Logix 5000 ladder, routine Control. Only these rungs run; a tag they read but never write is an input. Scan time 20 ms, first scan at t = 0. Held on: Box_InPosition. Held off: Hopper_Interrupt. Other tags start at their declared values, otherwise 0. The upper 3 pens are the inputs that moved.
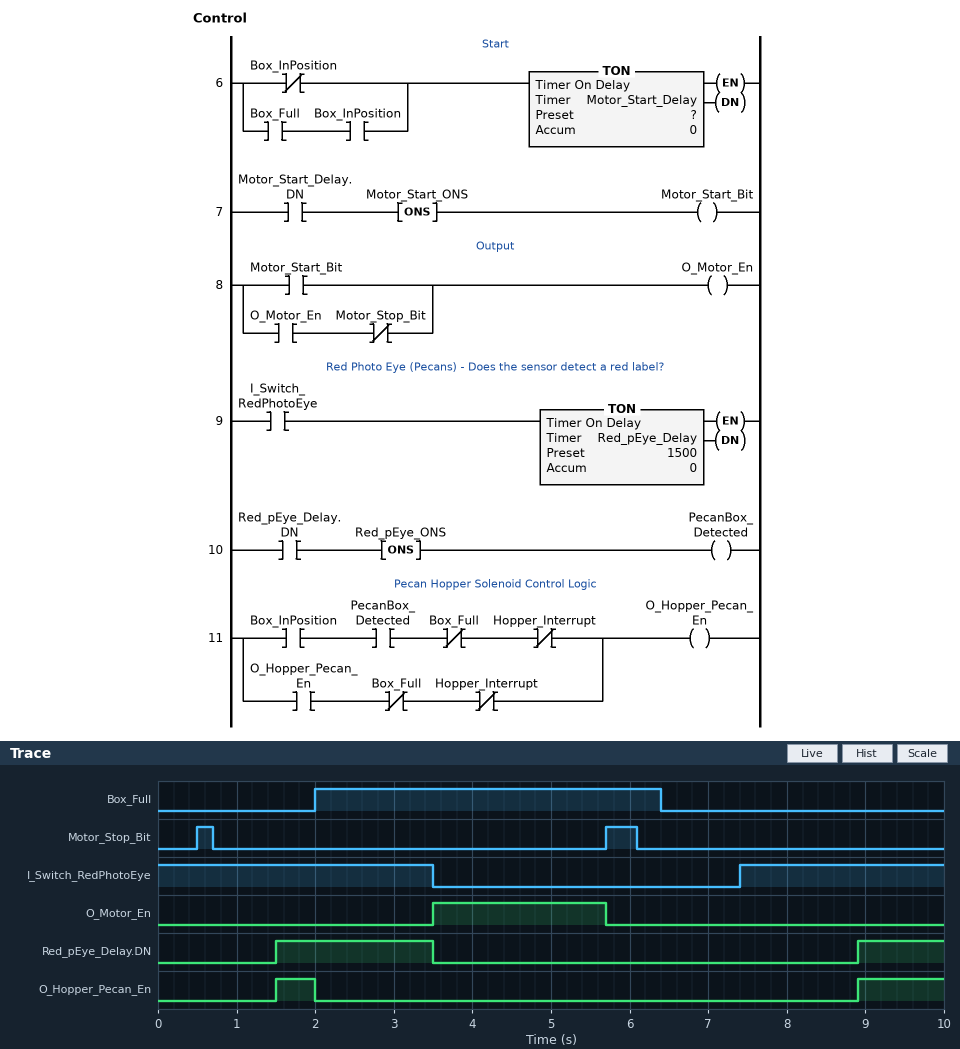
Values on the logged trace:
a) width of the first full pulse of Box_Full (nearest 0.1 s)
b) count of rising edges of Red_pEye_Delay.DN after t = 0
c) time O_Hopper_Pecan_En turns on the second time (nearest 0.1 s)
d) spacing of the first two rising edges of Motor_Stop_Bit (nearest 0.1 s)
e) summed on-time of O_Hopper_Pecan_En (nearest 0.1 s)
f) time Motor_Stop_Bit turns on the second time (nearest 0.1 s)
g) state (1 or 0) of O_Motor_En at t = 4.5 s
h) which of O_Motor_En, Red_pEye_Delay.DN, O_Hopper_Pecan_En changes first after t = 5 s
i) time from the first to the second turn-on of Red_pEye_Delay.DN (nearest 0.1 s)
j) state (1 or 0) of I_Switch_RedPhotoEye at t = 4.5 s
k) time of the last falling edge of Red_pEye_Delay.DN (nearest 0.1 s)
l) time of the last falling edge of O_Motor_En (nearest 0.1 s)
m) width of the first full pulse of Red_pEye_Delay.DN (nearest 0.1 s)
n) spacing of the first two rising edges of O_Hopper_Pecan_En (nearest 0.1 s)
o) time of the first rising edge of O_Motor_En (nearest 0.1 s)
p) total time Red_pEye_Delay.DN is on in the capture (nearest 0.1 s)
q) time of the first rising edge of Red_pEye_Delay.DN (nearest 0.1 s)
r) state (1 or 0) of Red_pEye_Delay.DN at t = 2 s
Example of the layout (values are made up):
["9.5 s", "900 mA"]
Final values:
["4.4 s", "2", "8.9 s", "5.2 s", "1.6 s", "5.7 s", "1", "O_Motor_En", "7.4 s", "0", "3.5 s", "5.7 s", "2.0 s", "7.4 s", "3.5 s", "3.1 s", "1.5 s", "1"]
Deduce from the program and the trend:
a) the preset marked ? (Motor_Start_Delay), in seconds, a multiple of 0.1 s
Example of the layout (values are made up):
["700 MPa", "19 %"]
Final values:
["1.5 s"]
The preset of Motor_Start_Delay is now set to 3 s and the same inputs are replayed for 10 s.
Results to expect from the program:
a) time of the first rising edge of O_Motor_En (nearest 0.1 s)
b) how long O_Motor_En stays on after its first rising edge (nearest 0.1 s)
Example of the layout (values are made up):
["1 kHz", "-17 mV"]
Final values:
["5.0 s", "0.7 s"]
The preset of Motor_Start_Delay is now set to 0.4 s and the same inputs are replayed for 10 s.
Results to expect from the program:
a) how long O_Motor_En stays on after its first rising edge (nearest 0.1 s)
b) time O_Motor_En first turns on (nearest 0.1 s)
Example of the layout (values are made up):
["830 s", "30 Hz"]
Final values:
["3.3 s", "2.4 s"]
